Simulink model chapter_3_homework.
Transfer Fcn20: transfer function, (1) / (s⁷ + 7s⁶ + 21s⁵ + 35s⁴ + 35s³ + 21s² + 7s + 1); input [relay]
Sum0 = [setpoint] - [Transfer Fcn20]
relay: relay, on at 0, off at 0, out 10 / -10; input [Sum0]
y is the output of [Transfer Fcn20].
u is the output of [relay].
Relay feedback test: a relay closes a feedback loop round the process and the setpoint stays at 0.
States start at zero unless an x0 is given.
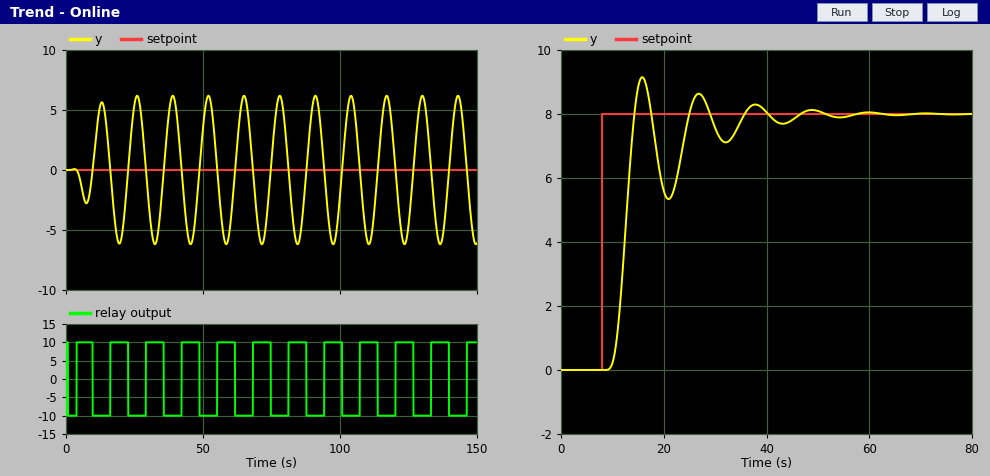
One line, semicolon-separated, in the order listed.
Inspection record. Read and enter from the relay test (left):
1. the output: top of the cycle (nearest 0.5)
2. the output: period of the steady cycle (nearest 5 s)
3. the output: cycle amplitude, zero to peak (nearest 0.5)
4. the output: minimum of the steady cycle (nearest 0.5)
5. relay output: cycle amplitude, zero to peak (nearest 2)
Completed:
6.0; 15 s; 6.0; -6.0; 10
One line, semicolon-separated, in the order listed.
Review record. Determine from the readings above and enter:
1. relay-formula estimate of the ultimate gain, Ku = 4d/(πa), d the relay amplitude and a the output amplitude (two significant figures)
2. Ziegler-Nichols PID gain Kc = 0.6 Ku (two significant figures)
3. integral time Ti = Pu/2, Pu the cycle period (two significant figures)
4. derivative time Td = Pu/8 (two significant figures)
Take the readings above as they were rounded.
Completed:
2.1; 1.3; 7.5 s; 1.9 s
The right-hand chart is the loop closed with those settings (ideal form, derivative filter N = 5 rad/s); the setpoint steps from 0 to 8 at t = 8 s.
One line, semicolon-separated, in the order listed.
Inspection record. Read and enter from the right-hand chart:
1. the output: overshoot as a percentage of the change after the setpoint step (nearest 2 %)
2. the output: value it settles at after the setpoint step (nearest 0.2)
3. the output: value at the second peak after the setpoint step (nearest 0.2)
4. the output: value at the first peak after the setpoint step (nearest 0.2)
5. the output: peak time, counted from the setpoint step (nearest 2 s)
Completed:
14 %; 8.0; 8.6; 9.2; 8 s
